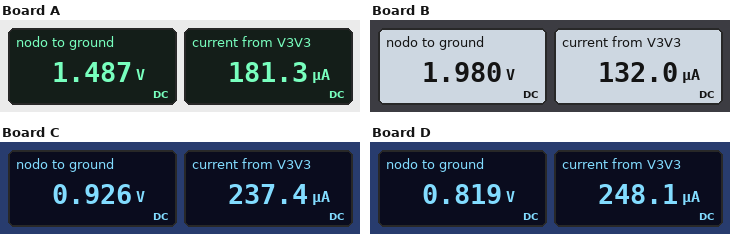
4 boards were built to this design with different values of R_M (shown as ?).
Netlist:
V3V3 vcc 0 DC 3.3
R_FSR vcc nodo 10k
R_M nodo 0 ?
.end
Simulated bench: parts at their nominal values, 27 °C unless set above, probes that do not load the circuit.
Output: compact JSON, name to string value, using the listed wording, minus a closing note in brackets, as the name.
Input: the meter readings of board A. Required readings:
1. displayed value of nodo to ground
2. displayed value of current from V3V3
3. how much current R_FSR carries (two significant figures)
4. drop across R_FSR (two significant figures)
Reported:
{"displayed value of nodo to ground": "1.487 V", "displayed value of current from V3V3": "181.3 µA", "how much current R_FSR carries": "180 µA", "drop across R_FSR": "1.8 V"}
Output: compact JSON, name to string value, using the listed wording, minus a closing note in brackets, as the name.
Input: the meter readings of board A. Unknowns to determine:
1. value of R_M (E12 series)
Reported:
{"value of R_M": "8.2 kΩ"}
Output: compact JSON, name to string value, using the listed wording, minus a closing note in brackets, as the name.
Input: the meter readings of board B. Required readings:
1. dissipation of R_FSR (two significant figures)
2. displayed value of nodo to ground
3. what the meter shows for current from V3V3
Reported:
{"dissipation of R_FSR": "170 µW", "displayed value of nodo to ground": "1.980 V", "what the meter shows for current from V3V3": "132.0 µA"}
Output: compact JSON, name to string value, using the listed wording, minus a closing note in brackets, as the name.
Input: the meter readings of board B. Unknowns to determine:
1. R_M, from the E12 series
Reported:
{"R_M, from the E12 series": "15 kΩ"}
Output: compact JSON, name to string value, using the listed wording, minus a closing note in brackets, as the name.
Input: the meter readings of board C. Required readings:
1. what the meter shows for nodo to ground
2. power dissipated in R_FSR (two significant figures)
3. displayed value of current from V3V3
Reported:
{"what the meter shows for nodo to ground": "0.926 V", "power dissipated in R_FSR": "560 µW", "displayed value of current from V3V3": "237.4 µA"}
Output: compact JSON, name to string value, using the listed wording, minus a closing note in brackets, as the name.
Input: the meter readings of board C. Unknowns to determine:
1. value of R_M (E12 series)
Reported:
{"value of R_M": "3.9 kΩ"}
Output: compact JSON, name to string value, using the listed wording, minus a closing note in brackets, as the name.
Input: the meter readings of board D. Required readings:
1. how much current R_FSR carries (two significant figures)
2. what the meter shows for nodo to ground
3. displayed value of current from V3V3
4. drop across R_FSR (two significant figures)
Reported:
{"how much current R_FSR carries": "250 µA", "what the meter shows for nodo to ground": "0.819 V", "displayed value of current from V3V3": "248.1 µA", "drop across R_FSR": "2.5 V"}
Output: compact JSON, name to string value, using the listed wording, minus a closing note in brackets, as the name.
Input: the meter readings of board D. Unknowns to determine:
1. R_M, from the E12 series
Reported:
{"R_M, from the E12 series": "3.3 kΩ"}
